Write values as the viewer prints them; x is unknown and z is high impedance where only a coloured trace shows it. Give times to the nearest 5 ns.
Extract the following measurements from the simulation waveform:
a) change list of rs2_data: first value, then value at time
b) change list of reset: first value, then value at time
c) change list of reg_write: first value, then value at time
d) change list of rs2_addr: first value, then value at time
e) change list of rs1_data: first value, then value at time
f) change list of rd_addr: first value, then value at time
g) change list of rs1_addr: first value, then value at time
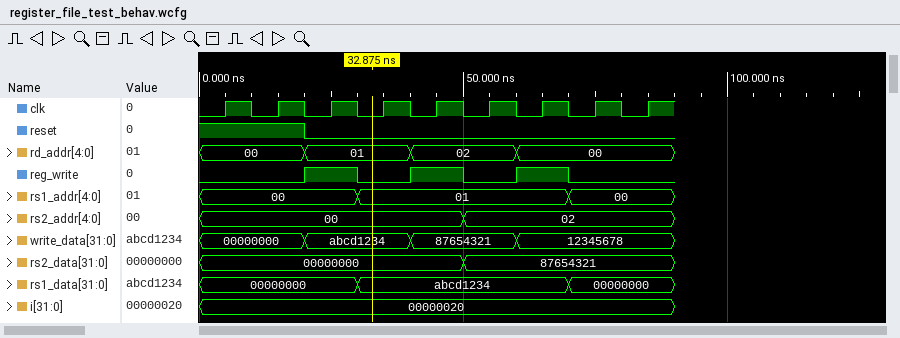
00000000, 87654321 at 50 ns
1, 0 at 20 ns
0, 1 at 20 ns, 0 at 30 ns, 1 at 40 ns, 0 at 50 ns, 1 at 60 ns, 0 at 70 ns
00, 02 at 50 ns
00000000, abcd1234 at 30 ns, 00000000 at 70 ns
00, 01 at 20 ns, 02 at 40 ns, 00 at 60 ns
00, 01 at 30 ns, 00 at 70 ns
